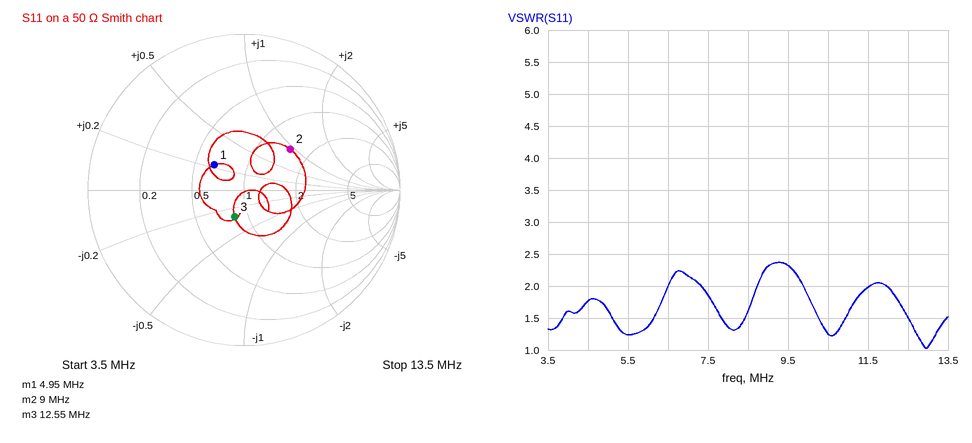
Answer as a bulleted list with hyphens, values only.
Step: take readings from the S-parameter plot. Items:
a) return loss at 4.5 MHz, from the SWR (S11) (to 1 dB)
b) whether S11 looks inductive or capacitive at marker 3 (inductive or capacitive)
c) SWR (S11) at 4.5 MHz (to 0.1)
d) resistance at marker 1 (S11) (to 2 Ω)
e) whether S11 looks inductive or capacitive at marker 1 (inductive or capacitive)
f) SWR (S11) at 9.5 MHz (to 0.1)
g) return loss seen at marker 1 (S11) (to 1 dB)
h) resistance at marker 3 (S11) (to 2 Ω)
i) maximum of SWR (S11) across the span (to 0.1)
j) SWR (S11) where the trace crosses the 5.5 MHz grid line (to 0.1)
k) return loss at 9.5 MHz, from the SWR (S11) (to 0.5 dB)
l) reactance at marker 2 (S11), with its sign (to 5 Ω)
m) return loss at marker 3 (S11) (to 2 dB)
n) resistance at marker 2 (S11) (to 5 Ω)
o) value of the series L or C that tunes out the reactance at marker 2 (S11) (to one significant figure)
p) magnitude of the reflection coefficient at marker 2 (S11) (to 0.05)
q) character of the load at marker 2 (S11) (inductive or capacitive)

- 11 dB
- capacitive
- 1.8
- 32 Ω
- inductive
- 2.3
- 12 dB
- 42 Ω
- 2.4
- 1.2
- 8.0 dB
- +45 Ω
- 14 dB
- 75 Ω
- 400 pF
- 0.40
- inductive
